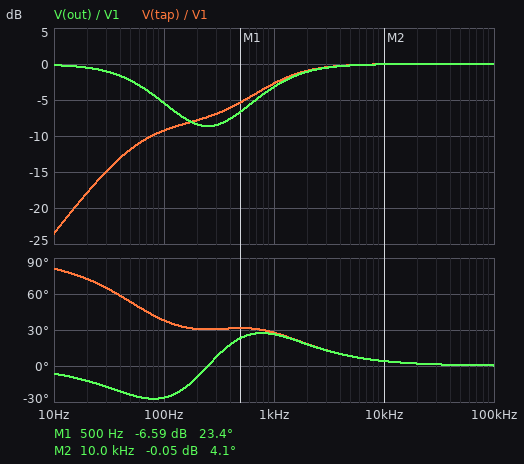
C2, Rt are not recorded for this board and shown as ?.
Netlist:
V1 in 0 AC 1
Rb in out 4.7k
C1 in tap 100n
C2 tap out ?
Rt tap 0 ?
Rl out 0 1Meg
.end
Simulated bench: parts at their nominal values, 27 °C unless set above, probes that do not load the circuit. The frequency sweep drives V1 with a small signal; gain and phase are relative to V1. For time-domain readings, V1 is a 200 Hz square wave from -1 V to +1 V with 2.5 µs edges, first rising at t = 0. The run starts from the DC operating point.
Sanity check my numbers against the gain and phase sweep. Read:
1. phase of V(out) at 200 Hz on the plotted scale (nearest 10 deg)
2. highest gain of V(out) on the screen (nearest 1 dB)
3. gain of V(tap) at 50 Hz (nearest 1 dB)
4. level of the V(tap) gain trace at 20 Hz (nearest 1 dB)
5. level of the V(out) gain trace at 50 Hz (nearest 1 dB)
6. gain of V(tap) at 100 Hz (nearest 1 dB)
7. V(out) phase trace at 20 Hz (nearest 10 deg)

-10 deg
0 dB
-12 dB
-18 dB
-2 dB
-9 dB
-10 deg
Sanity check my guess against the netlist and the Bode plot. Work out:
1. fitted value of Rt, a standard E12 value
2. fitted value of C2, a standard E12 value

2.2 kΩ
390 nF
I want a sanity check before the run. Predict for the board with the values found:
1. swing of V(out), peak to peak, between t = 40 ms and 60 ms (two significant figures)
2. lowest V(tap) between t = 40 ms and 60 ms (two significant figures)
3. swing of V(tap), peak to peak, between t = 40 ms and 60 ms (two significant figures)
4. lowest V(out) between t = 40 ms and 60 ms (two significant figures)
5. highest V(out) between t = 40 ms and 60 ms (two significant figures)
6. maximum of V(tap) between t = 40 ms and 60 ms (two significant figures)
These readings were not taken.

2.8 V
-1.8 V
3.6 V
-1.4 V
1.4 V
1.8 V
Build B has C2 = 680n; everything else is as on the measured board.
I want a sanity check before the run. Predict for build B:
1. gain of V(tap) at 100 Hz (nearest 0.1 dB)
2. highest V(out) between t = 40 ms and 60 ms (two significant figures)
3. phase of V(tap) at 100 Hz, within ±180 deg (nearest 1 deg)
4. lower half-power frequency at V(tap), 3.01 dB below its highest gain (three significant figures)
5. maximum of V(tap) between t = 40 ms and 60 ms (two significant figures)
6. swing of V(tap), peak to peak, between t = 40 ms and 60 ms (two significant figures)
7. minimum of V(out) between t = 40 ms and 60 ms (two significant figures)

-9.1 dB
1.5 V
28 deg
931 Hz
1.7 V
3.5 V
-1.5 V
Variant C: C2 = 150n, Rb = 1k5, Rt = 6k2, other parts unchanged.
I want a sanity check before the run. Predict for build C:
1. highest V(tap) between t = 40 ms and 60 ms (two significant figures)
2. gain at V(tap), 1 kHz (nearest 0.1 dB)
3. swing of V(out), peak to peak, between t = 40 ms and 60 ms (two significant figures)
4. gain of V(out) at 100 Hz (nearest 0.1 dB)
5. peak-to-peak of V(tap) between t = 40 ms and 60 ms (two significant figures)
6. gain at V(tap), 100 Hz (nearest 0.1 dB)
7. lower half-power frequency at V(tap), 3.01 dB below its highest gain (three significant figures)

1.7 V
-0.6 dB
2.1 V
-0.7 dB
3.3 V
-3.5 dB
114 Hz
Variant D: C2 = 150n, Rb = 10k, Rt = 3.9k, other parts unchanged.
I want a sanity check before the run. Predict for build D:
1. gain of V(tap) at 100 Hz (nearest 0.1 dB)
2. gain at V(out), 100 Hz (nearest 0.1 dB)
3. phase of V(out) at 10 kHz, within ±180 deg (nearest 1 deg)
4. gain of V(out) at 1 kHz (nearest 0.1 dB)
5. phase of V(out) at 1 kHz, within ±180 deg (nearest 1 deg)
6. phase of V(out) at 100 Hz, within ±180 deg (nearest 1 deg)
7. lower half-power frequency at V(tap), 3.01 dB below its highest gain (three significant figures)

-8.5 dB
-5.0 dB
2 deg
-1.4 dB
20 deg
-25 deg
486 Hz
